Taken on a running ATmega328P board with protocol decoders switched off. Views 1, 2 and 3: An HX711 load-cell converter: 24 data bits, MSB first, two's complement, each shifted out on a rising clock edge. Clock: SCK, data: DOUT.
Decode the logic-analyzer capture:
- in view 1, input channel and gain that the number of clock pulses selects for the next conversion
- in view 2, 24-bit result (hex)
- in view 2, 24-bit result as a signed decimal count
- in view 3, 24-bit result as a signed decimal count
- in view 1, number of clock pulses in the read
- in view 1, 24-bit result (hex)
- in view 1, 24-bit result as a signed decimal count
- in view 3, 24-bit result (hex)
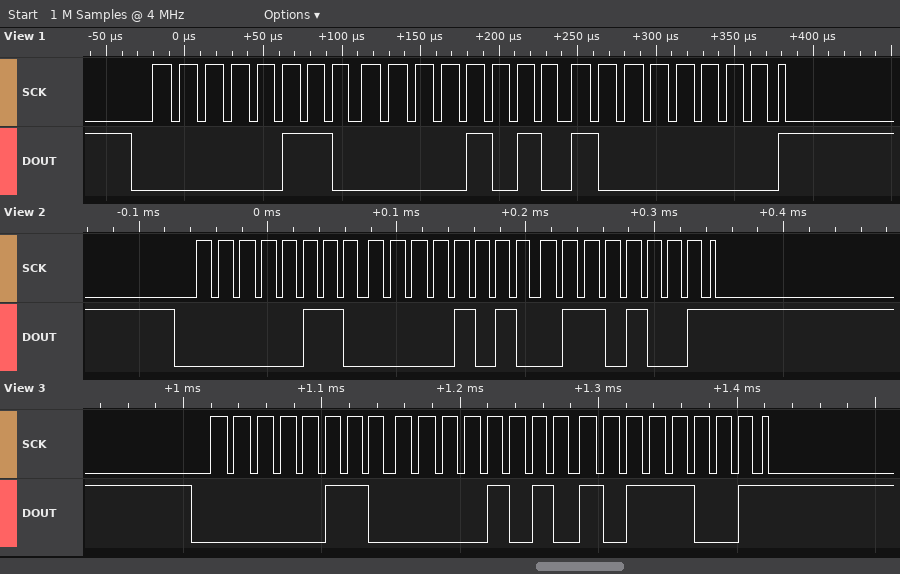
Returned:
channel A, gain 128
0x060A69
395881
395961
25
0x060A80
395904
0x060AB9
